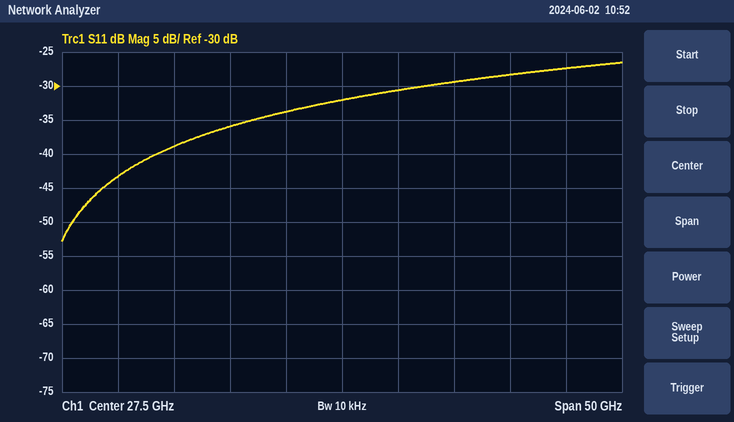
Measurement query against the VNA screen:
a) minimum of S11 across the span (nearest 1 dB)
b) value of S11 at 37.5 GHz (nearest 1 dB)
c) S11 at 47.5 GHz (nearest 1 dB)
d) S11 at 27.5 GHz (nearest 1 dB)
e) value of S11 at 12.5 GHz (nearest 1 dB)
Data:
-53 dB
-29 dB
-27 dB
-32 dB
-39 dB
